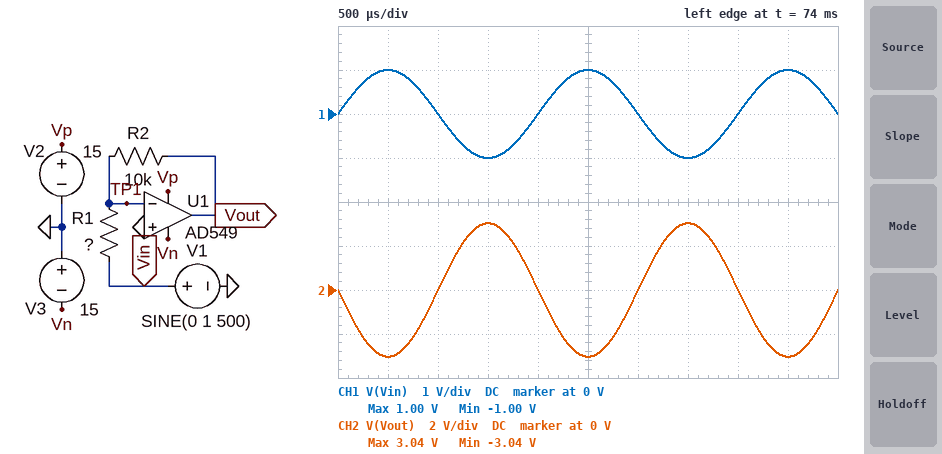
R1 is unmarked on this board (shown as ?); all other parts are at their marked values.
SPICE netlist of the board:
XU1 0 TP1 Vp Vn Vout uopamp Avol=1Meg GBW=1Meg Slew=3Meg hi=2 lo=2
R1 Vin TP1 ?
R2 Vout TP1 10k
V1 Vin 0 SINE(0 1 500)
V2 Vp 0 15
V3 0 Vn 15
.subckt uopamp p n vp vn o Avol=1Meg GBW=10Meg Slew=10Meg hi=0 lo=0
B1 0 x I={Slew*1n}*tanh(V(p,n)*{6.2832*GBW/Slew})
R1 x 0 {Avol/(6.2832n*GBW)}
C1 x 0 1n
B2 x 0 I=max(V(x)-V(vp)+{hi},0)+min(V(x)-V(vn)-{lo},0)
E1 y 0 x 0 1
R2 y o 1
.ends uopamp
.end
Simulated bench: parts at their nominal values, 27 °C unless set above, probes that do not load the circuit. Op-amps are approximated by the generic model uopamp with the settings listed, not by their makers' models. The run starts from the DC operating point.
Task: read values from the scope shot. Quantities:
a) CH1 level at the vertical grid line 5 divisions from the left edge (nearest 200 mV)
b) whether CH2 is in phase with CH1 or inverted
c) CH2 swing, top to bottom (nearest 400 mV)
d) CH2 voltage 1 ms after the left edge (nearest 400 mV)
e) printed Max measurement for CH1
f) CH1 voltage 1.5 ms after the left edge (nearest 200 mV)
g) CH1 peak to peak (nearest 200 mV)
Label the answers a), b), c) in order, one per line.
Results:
a) 1.0 V
b) inverted
c) 6.0 V
d) 0 V
e) 1.00 V
f) -1.0 V
g) 2.0 V
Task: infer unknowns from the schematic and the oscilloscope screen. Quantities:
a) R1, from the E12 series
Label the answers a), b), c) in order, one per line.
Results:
a) 3.3 kΩ
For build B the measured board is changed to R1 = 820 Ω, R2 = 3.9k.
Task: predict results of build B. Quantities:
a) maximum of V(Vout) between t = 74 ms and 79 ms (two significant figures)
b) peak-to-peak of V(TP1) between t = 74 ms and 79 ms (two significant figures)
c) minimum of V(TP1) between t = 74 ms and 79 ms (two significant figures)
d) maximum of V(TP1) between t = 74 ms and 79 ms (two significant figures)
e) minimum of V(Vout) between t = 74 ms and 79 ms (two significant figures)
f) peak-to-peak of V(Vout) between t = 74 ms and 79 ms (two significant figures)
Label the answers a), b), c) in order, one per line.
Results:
a) 4.8 V
b) 4.8 mV
c) -2.4 mV
d) 2.4 mV
e) -4.8 V
f) 9.5 V
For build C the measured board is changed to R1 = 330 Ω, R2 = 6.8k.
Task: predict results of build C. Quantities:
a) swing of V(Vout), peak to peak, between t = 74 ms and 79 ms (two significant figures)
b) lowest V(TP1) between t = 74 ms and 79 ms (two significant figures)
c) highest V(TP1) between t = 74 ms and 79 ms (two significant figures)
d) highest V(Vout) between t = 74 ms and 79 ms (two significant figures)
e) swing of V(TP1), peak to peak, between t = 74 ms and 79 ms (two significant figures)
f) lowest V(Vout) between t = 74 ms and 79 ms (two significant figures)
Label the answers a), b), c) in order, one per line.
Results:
a) 26 V
b) -350 mV
c) 350 mV
d) 13 V
e) 700 mV
f) -13 V
